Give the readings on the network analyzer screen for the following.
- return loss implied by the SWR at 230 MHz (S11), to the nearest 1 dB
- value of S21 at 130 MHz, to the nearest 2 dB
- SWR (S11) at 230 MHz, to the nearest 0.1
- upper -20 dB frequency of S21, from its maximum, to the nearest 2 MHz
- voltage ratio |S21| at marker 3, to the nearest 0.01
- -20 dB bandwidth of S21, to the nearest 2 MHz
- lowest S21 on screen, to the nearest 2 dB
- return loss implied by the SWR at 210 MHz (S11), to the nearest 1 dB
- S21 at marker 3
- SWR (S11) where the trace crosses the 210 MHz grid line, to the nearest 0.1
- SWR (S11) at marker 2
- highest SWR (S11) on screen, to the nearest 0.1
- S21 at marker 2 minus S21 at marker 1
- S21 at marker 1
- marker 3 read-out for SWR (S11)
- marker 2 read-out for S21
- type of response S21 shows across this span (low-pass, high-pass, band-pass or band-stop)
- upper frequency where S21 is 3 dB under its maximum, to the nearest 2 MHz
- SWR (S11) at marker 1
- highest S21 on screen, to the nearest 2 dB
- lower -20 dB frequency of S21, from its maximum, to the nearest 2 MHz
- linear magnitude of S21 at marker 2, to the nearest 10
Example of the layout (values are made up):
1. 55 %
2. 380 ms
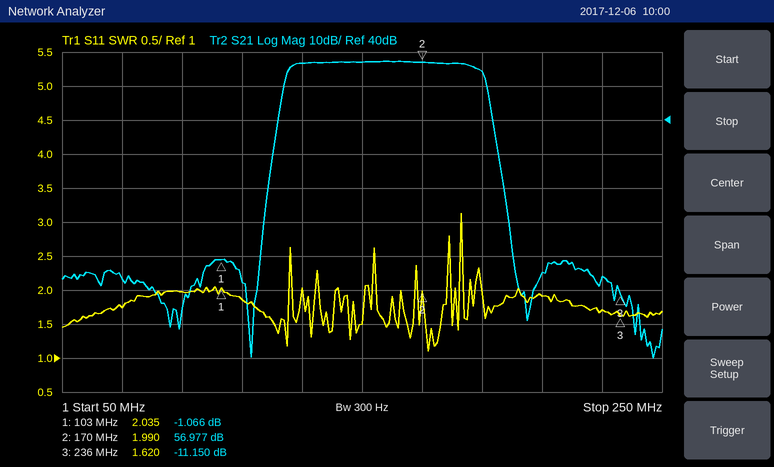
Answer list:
1. 12 dB
2. 56 dB
3. 1.7
4. 194 MHz
5. 0.28
6. 72 MHz
7. -30 dB
8. 10 dB
9. -11.150 dB
10. 1.9
11. 1.990
12. 3.1
13. 58.043 dB
14. -1.066 dB
15. 1.620
16. 56.977 dB
17. band-pass
18. 190 MHz
19. 2.035
20. 58 dB
21. 122 MHz
22. 710
